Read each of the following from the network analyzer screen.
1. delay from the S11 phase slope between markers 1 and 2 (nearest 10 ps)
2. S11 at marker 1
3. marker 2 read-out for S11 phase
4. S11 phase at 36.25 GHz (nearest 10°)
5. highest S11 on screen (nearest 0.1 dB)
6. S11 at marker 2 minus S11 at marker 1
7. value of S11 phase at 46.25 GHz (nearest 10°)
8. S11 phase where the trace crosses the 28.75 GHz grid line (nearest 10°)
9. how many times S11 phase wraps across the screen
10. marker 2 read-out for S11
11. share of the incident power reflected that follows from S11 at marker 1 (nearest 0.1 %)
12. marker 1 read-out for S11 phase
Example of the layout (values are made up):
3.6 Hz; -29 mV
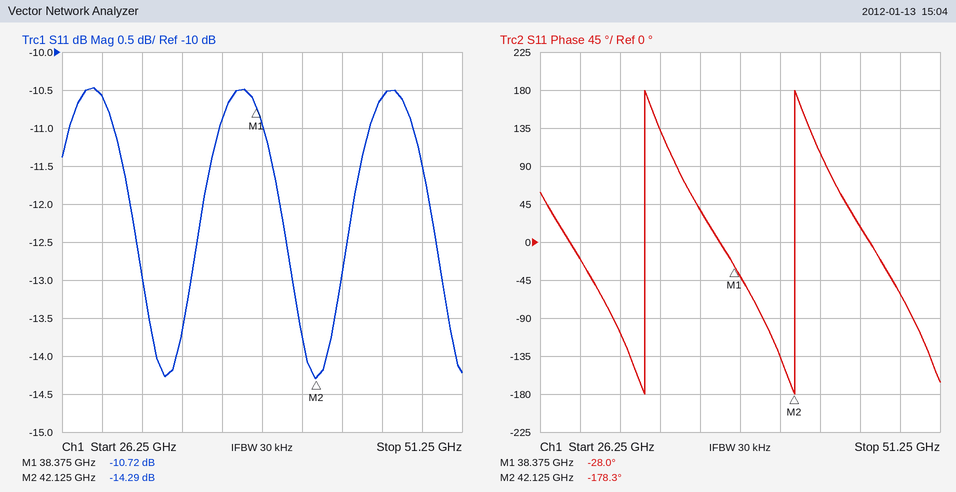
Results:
110 ps; -10.72 dB; -178.3°; 40°; -10.5 dB; -3.57 dB; 20°; -20°; 2; -14.29 dB; 8.5 %; -28.0°
